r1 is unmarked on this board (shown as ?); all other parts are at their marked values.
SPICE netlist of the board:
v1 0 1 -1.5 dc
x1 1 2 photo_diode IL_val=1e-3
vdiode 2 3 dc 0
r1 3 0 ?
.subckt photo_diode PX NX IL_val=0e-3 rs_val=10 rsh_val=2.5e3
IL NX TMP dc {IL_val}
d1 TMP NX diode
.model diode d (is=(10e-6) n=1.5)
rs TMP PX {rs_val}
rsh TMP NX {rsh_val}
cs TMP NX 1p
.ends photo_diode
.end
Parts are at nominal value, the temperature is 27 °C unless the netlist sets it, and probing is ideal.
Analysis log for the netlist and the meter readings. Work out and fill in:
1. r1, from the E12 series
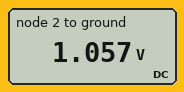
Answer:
68 Ω
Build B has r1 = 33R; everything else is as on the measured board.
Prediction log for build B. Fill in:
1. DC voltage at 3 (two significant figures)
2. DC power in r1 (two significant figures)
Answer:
910 mV
25 mW
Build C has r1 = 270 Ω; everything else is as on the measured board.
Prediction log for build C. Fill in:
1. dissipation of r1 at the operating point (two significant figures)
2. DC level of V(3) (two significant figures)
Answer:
5.4 mW
1.2 V
